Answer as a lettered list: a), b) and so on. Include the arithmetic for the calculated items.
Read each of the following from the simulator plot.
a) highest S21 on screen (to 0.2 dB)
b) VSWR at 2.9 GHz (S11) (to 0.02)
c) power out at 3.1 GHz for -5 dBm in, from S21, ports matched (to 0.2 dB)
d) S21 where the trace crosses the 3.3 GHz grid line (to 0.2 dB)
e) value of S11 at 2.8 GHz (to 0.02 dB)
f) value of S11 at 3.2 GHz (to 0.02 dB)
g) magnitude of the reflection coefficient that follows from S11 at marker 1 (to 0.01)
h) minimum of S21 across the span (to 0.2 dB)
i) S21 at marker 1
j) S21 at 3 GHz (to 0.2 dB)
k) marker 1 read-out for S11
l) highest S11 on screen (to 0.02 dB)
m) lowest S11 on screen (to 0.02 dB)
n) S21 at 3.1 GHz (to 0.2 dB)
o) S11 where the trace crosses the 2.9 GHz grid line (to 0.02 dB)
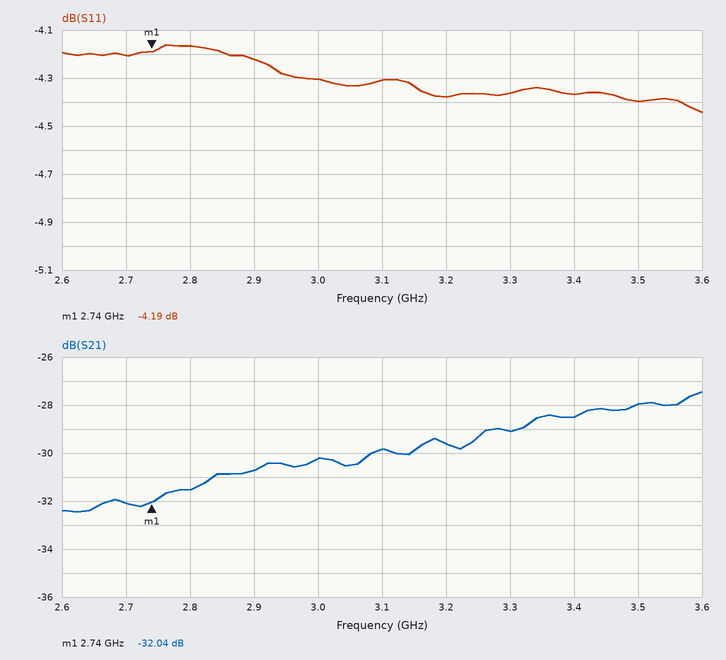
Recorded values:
a) -27.4 dB
b) |Γ| = 10^(-4.22/20) = 0.6152; VSWR = (1 + 0.6152)/(1 − 0.6152) ≈ 4.20
c) -5 dBm + (-29.8 dB) = -34.8 dBm
d) -29.0 dB
e) -4.16 dB
f) -4.38 dB
g) 10^(-4.19/20) ≈ 0.62
h) -32.4 dB
i) -32.04 dB
j) -30.2 dB
k) -4.19 dB
l) -4.16 dB
m) -4.44 dB
n) -29.8 dB
o) -4.22 dB
